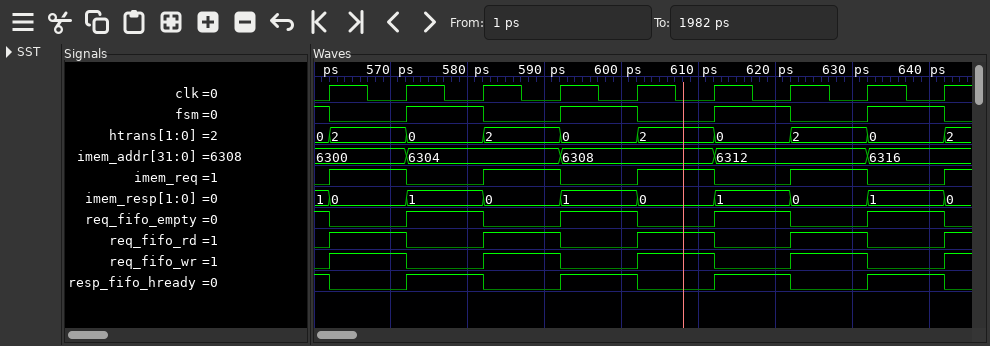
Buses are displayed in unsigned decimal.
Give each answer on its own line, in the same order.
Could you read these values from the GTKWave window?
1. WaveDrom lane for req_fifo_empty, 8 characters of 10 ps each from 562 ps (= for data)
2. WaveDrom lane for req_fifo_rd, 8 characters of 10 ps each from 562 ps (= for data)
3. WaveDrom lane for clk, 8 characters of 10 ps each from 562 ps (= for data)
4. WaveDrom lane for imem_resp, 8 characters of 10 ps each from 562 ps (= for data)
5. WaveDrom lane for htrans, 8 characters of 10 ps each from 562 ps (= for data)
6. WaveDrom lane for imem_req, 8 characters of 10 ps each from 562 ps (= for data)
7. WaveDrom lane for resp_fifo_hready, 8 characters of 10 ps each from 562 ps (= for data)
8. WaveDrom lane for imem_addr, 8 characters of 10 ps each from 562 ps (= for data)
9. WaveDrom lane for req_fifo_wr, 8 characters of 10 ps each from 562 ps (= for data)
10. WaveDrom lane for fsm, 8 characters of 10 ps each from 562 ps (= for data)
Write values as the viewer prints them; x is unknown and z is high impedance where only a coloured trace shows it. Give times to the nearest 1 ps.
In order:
{name: 'req_fifo_empty', wave: '01010101'}
{name: 'req_fifo_rd', wave: '10101010'}
{name: 'clk', wave: 'p.......'}
{name: 'imem_resp', wave: '========', data: '0 1 0 1 0 1 0 1'}
{name: 'htrans', wave: '========', data: '2 0 2 0 2 0 2 0'}
{name: 'imem_req', wave: '10101010'}
{name: 'resp_fifo_hready', wave: '01010101'}
{name: 'imem_addr', wave: '==.=.=.=', data: '6300 6304 6308 6312 6316'}
{name: 'req_fifo_wr', wave: '10101010'}
{name: 'fsm', wave: '01010101'}
